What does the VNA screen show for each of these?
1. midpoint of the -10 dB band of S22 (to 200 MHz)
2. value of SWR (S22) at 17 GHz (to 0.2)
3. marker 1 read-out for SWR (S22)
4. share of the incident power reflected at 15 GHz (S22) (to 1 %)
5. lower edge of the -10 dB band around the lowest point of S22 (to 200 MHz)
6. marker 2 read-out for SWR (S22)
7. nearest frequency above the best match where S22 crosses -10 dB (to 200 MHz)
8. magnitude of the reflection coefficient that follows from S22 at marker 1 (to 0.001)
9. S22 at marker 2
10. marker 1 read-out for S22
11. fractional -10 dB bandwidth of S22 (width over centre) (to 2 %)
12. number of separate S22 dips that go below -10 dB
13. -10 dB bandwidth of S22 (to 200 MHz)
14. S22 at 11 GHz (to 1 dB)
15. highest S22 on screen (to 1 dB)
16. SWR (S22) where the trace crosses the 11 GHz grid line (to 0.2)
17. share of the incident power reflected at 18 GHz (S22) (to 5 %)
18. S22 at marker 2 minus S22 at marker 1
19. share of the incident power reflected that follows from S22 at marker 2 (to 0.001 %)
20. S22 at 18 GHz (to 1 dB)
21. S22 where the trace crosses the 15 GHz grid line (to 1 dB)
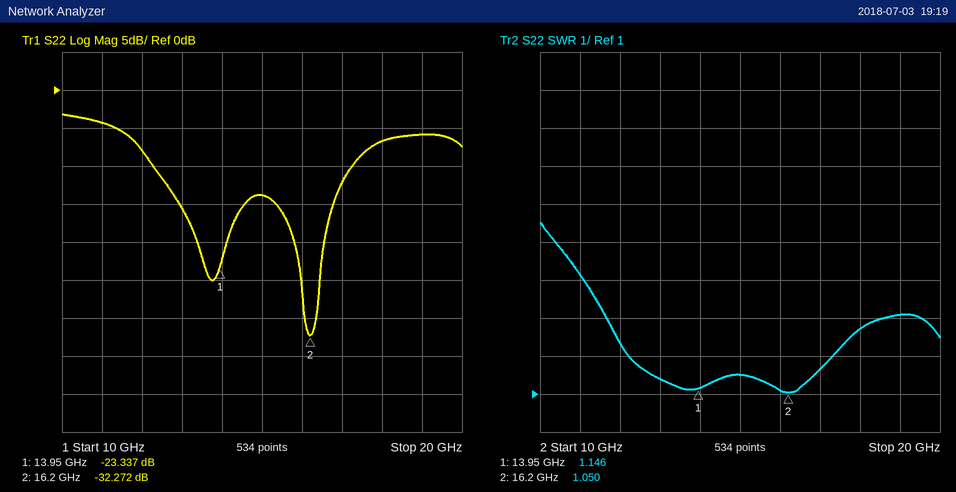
14.8 GHz
1.6
1.146
4 %
12.2 GHz
1.050
17.2 GHz
0.068
-32.272 dB
-23.337 dB
34 %
2
5.0 GHz
-4 dB
-3 dB
4.2
20 %
-8.935 dB
0.059 %
-7 dB
-14 dB
